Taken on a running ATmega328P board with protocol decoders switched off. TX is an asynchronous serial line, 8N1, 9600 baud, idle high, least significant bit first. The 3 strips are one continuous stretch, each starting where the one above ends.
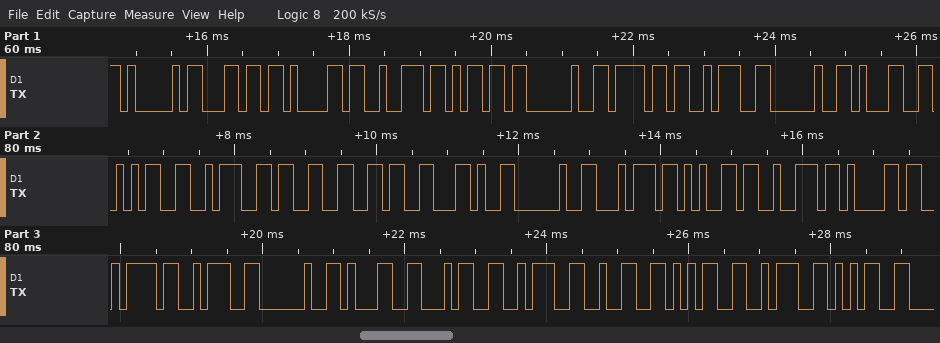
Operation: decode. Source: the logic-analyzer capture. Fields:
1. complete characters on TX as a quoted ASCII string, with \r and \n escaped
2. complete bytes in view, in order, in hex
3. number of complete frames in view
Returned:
"Alarm o: 15:36, teraz: 14:25:5"
41 6C 61 72 6D 20 6F 3A 20 31 35 3A 33 36 2C 20 74 65 72 61 7A 3A 20 31 34 3A 32 35 3A 35
30
